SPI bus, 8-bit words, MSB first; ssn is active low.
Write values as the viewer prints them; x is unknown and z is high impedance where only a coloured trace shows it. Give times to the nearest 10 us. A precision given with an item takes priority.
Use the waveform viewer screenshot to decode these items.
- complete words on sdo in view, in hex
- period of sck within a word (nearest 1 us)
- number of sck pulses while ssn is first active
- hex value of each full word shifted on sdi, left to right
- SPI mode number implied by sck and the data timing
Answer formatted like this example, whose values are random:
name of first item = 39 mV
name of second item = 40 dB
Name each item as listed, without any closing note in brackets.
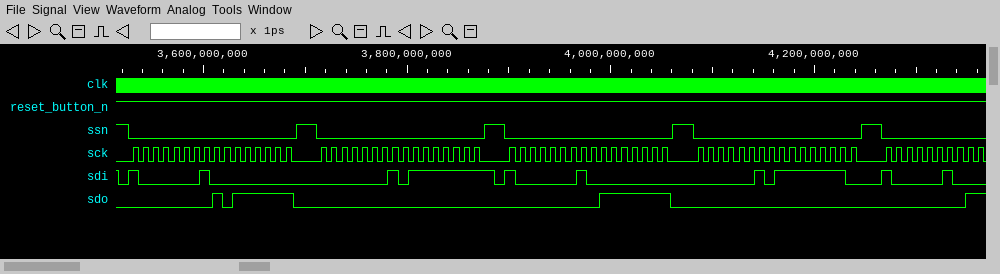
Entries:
complete words on sdo in view, in hex = 00, BF, 00, 00, 00, 7F, 00, 00, 00
period of sck within a word = 10 us
number of sck pulses while ssn is first active = 16
hex value of each full word shifted on sdi, left to right = 81, 00, 01, 7F, 81, 00, 02, FE, 82
SPI mode number implied by sck and the data timing = 0
